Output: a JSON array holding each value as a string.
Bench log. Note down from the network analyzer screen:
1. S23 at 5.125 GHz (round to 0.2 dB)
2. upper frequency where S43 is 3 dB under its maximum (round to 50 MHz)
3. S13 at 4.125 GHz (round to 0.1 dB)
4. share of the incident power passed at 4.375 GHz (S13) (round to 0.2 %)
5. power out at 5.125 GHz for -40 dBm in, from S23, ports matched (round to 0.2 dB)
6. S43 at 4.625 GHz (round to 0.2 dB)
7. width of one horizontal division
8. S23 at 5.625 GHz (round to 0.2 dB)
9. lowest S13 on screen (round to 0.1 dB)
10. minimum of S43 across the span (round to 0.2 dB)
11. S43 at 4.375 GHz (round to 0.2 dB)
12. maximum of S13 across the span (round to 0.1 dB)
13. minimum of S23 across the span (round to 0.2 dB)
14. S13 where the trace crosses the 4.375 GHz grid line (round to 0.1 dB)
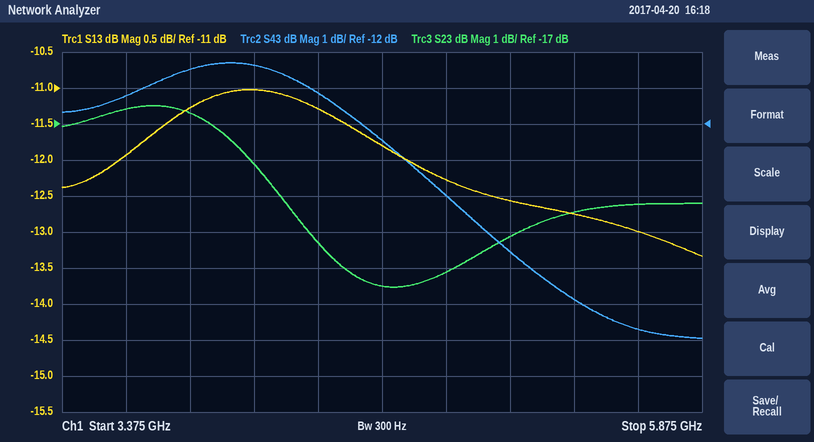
["-20.2 dB", "4.75 GHz", "-11.0 dB", "7.4 %", "-60.2 dBm", "-12.4 dB", "250 MHz", "-19.2 dB", "-13.3 dB", "-18.0 dB", "-11.2 dB", "-11.0 dB", "-21.6 dB", "-11.3 dB"]
